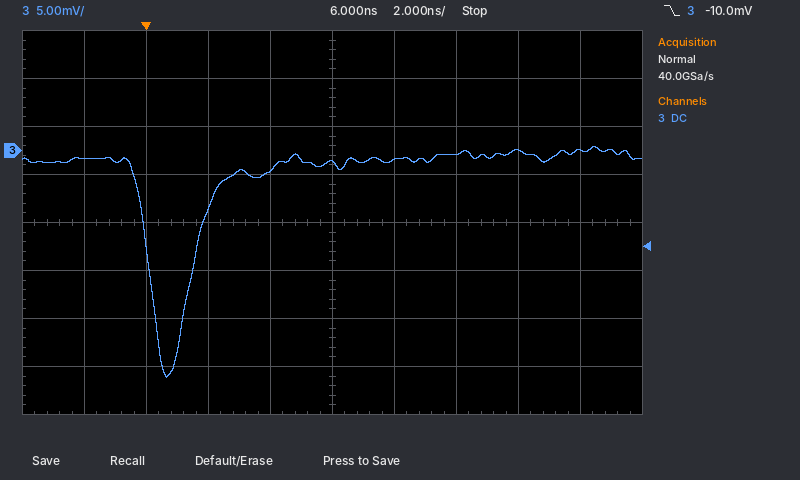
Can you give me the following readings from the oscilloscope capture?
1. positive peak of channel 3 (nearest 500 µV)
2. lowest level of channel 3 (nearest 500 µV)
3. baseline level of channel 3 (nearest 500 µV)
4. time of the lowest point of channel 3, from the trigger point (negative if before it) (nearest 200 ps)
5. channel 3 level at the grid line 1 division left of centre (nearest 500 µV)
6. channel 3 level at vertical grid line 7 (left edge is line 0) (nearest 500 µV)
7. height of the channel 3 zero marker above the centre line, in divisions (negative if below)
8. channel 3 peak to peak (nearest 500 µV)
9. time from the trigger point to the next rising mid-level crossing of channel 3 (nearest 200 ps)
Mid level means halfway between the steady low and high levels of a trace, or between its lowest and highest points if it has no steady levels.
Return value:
500 µV
-23.5 mV
-1.0 mV
+600 ps
-2.0 mV
-500 µV
+1.5 div
24.0 mV
1.6 ns
